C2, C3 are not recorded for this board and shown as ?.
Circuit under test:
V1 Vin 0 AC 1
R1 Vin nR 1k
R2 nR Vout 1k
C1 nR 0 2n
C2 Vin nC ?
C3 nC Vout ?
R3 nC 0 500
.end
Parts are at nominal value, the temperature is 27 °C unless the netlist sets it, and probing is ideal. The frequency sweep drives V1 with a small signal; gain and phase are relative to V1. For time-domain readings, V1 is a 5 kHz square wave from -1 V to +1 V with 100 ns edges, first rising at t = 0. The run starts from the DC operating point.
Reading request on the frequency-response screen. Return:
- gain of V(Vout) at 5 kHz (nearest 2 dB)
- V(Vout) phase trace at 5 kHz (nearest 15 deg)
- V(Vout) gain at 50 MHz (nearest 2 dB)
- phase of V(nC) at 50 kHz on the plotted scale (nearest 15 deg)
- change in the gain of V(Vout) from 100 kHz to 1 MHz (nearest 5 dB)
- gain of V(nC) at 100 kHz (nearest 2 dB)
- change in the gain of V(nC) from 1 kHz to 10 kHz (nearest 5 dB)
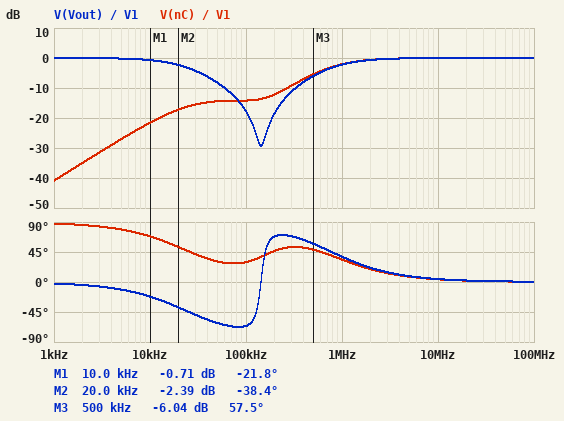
0 dB
-15 deg
0 dB
30 deg
15 dB
-14 dB
20 dB
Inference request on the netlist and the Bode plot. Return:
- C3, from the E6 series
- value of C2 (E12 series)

2.2 nF
680 pF
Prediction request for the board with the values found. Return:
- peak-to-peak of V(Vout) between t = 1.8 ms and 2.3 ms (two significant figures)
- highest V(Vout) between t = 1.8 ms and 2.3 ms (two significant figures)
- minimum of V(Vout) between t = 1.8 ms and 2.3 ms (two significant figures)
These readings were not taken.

2.0 V
1.0 V
-1.0 V
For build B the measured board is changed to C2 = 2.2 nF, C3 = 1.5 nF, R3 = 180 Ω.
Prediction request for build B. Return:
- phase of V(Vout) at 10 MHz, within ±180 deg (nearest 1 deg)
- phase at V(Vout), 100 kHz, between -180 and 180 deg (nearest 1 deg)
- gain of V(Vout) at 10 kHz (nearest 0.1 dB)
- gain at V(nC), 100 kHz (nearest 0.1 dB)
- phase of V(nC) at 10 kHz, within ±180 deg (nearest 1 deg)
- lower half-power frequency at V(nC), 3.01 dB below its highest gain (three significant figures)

3 deg
-97 deg
-0.4 dB
-12.8 dB
81 deg
507 kHz
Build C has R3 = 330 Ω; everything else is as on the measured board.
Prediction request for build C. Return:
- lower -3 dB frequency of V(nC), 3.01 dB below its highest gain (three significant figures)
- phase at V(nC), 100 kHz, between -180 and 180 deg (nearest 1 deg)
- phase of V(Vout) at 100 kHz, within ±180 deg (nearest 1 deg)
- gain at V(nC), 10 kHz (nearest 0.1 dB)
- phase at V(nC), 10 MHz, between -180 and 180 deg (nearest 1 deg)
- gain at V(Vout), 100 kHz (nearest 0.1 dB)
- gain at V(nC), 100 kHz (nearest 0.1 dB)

1.01 MHz
35 deg
-83 deg
-25.1 dB
5 deg
-16.6 dB
-17.1 dB
